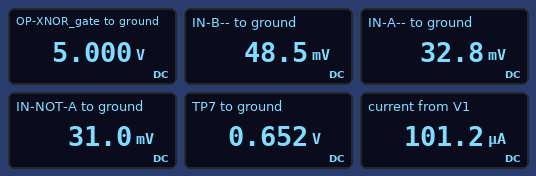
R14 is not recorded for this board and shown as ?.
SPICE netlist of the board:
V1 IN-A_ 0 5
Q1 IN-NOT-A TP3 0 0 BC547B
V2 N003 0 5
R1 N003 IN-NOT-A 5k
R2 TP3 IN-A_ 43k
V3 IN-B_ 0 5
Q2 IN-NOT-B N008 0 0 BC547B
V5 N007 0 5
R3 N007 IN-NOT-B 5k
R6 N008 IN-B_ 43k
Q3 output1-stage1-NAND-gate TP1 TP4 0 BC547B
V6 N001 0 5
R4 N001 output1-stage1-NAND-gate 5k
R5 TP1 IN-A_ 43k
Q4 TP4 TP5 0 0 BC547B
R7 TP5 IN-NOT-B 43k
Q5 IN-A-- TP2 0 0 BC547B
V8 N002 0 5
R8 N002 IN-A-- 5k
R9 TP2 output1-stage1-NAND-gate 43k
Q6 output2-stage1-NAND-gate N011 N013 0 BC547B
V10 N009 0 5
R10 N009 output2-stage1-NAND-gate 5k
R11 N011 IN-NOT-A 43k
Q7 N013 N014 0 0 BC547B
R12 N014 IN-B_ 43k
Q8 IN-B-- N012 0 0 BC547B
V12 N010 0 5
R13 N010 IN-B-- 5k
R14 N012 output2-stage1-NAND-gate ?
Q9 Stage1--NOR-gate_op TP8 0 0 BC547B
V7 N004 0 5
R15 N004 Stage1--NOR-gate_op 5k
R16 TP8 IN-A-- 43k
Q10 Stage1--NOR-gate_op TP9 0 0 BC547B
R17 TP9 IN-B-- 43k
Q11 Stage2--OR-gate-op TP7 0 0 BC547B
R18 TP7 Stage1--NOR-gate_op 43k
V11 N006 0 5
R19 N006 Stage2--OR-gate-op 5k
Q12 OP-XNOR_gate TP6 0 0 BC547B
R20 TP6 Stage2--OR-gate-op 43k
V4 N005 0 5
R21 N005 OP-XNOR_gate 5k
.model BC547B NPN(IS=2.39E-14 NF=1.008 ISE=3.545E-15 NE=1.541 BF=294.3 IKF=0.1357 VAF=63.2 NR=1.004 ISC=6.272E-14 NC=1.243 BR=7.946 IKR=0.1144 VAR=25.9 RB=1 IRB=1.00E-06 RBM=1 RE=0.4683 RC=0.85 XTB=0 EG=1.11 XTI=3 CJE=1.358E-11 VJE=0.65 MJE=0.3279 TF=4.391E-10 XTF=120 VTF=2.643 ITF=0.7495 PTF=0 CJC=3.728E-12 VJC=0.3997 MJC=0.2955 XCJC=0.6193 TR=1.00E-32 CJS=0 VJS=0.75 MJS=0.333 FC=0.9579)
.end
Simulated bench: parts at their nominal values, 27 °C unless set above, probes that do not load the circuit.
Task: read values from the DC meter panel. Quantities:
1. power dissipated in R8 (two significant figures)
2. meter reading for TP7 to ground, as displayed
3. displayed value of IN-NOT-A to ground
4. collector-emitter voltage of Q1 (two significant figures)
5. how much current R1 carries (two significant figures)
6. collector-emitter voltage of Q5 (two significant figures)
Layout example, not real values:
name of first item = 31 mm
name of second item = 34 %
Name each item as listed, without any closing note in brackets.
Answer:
power dissipated in R8 = 4.9 mW
meter reading for TP7 to ground, as displayed = 0.652 V
displayed value of IN-NOT-A to ground = 31.0 mV
collector-emitter voltage of Q1 = 31 mV
how much current R1 carries = 990 µA
collector-emitter voltage of Q5 = 33 mV
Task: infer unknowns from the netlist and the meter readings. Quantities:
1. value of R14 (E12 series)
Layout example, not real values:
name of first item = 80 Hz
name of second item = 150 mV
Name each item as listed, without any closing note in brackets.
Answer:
value of R14 = 100 kΩ
